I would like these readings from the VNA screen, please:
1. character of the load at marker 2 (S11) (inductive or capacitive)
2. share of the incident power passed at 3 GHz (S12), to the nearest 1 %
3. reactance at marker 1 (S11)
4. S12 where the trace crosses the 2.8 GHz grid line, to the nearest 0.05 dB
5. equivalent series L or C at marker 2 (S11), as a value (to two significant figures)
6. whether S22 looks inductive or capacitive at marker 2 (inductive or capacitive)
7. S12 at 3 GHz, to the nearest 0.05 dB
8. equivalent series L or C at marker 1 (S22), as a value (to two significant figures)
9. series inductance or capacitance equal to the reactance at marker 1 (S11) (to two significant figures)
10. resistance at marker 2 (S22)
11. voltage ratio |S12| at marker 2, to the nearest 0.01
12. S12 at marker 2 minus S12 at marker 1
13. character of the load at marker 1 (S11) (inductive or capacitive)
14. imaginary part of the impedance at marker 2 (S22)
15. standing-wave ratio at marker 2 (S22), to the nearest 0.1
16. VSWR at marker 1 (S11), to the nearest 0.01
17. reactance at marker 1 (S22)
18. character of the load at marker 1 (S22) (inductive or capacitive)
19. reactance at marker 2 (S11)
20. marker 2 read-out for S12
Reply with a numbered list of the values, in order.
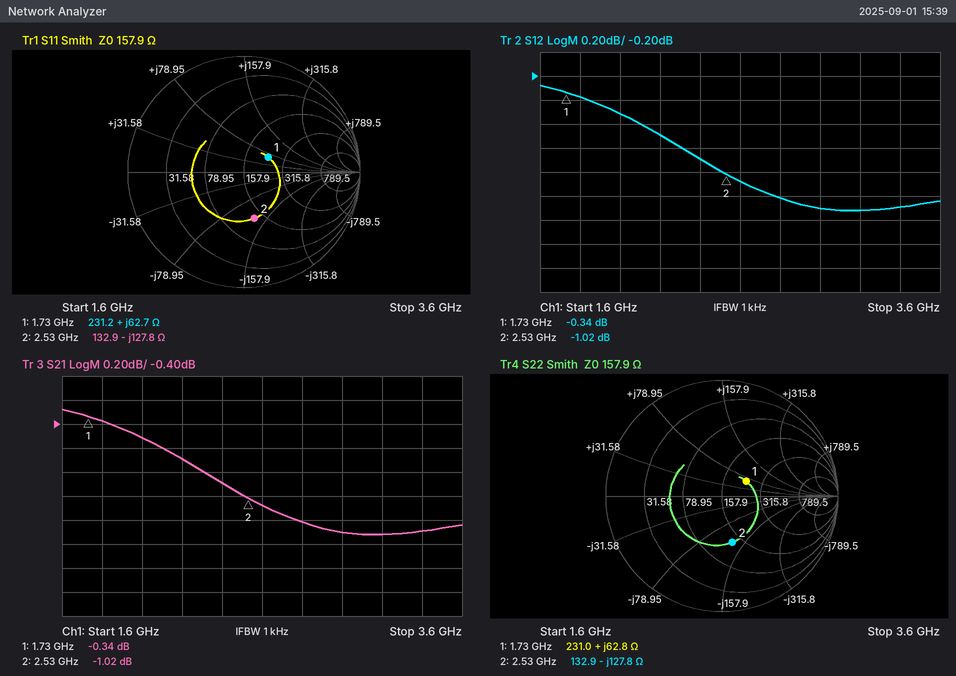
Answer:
1. capacitive
2. 74 %
3. +62.7 Ω
4. -1.20 dB
5. 490 fF
6. capacitive
7. -1.30 dB
8. 5.8 nH
9. 5.8 nH
10. 132.9 Ω
11. 0.89
12. -0.68 dB
13. inductive
14. -127.8 Ω
15. 2.4
16. 1.65
17. +62.8 Ω
18. inductive
19. -127.8 Ω
20. -1.02 dB
